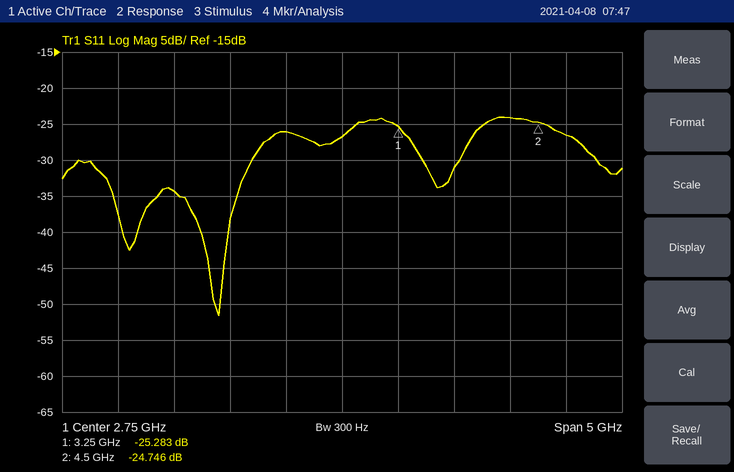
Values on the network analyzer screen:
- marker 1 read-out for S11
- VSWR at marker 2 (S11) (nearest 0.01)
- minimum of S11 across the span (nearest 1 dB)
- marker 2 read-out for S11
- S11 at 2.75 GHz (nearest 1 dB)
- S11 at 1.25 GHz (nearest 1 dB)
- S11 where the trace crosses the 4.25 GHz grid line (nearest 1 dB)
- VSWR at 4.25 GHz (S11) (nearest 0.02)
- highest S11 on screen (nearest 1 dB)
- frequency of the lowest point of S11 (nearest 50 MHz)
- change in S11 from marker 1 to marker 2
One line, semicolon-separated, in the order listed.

-25.283 dB; 1.12; -52 dB; -24.746 dB; -27 dB; -34 dB; -24 dB; 1.14; -24 dB; 1.65 GHz; 0.537 dB
